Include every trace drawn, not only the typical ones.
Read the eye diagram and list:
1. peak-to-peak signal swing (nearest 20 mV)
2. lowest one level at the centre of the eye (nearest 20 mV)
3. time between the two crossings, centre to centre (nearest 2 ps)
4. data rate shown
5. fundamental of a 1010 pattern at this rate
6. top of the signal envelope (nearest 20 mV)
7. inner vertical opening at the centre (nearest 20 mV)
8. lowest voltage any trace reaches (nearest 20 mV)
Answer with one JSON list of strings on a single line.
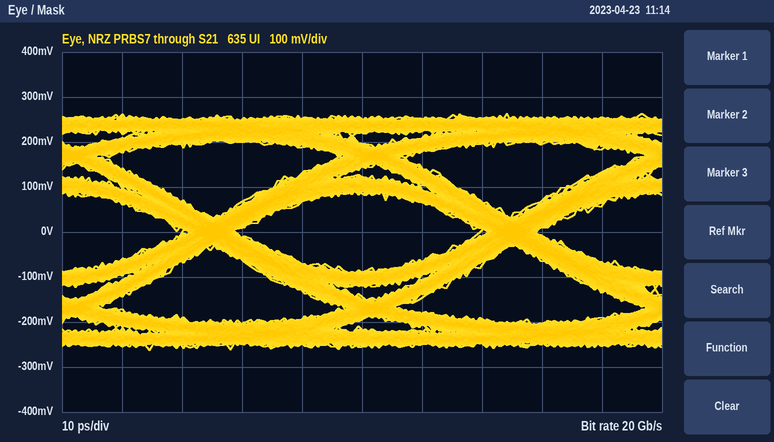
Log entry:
["520 mV", "80 mV", "50 ps", "20 Gb/s", "10 GHz", "260 mV", "180 mV", "-260 mV"]
